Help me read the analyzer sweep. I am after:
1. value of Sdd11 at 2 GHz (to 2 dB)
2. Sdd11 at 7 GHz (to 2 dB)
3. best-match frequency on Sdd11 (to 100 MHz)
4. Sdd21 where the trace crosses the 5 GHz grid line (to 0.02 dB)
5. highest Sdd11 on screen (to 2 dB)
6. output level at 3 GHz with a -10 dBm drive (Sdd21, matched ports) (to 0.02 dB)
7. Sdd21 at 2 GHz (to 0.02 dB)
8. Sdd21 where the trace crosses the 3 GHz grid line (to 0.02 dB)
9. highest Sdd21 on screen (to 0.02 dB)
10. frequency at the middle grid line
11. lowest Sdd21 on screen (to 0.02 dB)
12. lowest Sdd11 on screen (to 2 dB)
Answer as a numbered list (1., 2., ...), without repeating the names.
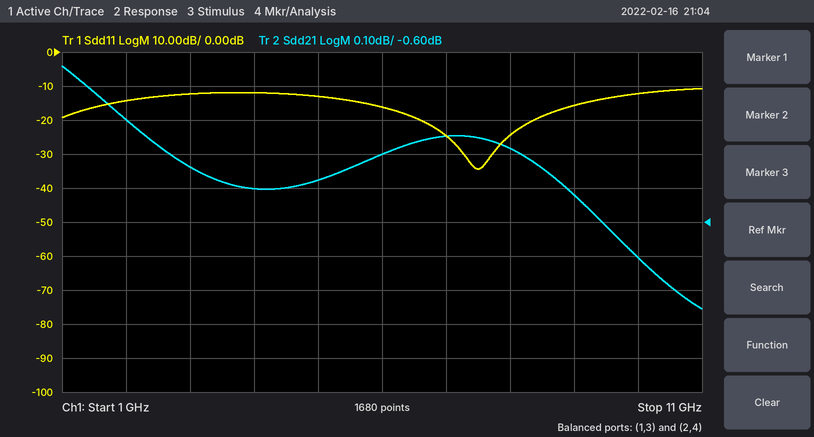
1. -14 dB
2. -24 dB
3. 7.5 GHz
4. -0.48 dB
5. -10 dB
6. -10.44 dBm
7. -0.30 dB
8. -0.44 dB
9. -0.14 dB
10. 6 GHz
11. -0.86 dB
12. -34 dB
